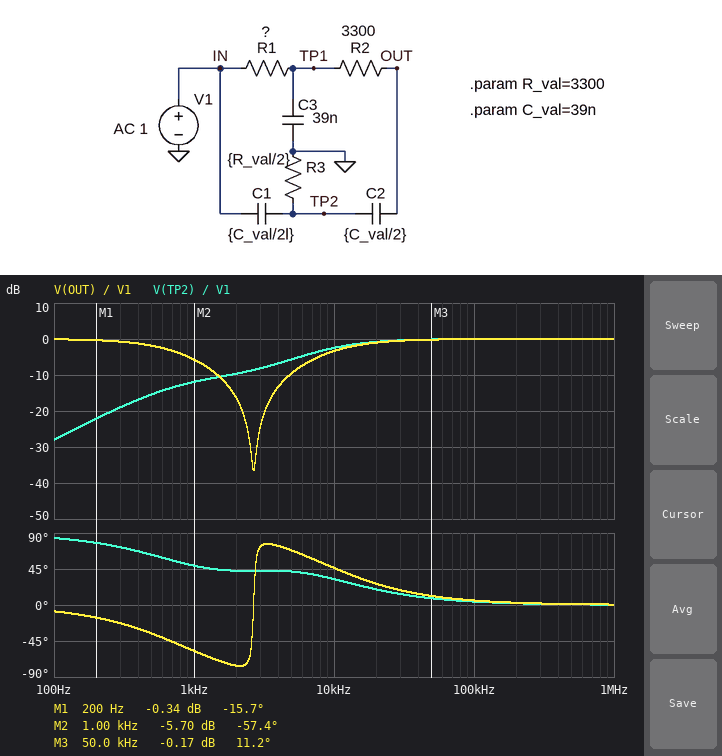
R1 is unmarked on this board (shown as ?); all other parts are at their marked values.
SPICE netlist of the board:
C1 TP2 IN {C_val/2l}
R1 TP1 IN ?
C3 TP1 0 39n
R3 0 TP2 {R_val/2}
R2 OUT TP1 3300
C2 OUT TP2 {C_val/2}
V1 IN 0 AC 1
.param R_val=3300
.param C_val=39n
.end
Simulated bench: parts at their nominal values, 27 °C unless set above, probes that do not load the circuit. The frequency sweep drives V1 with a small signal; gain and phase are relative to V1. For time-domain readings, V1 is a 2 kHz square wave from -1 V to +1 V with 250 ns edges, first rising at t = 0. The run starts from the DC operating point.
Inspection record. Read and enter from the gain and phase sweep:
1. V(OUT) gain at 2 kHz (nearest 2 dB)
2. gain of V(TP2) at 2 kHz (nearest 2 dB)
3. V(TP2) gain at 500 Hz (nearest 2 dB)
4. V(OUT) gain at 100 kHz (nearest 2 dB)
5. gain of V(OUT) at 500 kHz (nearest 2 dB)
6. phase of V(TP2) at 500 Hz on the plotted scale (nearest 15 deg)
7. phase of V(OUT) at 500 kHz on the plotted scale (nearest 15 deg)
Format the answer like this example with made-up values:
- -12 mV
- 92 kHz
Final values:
- -16 dB
- -10 dB
- -16 dB
- 0 dB
- 0 dB
- 60 deg
- 0 deg
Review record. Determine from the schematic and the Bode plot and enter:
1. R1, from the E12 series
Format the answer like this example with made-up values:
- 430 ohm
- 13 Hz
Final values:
- 2.7 kΩ
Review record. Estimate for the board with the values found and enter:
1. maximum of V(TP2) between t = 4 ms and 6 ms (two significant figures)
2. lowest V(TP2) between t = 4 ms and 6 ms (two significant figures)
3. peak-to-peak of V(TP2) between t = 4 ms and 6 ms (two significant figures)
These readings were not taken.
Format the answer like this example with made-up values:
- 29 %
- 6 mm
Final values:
- 1.9 V
- -1.9 V
- 3.7 V
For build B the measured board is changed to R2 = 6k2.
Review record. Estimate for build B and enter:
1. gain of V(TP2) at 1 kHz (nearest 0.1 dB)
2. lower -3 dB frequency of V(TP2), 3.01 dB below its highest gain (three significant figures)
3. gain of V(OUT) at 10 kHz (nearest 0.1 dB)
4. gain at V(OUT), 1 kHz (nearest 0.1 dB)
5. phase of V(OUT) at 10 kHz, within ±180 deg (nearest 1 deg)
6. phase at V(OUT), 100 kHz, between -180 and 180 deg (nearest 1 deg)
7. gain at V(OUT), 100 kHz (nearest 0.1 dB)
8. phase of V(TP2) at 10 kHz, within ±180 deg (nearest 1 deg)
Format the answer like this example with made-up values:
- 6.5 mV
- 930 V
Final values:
- -12.9 dB
- 6.99 kHz
- -2.1 dB
- -7.8 dB
- 39 deg
- 4 deg
- 0 dB
- 31 deg
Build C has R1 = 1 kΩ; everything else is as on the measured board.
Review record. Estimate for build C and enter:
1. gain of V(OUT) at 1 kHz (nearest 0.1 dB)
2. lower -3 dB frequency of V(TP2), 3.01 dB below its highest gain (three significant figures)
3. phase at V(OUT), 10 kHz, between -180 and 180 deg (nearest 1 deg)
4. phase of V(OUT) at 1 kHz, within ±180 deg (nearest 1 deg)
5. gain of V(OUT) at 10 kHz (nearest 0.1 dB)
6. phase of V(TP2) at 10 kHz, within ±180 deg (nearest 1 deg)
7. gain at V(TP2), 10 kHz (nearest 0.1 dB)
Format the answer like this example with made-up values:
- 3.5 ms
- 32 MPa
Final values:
- -2.8 dB
- 9.30 kHz
- 43 deg
- -36 deg
- -4.3 dB
- 30 deg
- -2.7 dB
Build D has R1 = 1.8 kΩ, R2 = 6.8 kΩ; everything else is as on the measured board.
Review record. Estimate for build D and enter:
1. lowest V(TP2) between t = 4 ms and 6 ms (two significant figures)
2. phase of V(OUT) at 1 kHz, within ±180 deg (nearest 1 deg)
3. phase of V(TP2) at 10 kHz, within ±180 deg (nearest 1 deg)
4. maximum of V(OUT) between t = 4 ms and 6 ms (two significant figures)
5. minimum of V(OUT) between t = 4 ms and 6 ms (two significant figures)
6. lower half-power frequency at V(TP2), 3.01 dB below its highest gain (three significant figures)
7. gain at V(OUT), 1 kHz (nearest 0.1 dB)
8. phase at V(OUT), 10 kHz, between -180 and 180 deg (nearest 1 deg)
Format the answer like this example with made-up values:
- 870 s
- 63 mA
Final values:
- -1.9 V
- -60 deg
- 30 deg
- 1.6 V
- -1.6 V
- 6.97 kHz
- -6.7 dB
- 37 deg
